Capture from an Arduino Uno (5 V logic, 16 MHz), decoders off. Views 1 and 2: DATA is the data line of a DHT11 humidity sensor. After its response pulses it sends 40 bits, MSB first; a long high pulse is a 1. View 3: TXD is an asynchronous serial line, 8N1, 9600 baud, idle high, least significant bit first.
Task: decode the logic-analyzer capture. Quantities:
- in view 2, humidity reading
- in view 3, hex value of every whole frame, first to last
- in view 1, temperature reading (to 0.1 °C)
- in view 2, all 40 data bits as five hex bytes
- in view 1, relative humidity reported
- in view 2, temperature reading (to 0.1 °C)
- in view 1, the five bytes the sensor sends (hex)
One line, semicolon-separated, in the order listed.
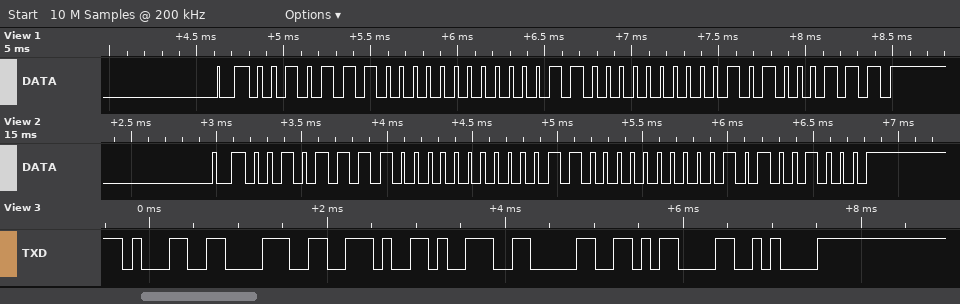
47 %; 31 38 2E 39 30 0D 0A; 24.1 °C; 2F 00 18 01 48; 46 %; 24.1 °C; 2E 00 18 01 47
